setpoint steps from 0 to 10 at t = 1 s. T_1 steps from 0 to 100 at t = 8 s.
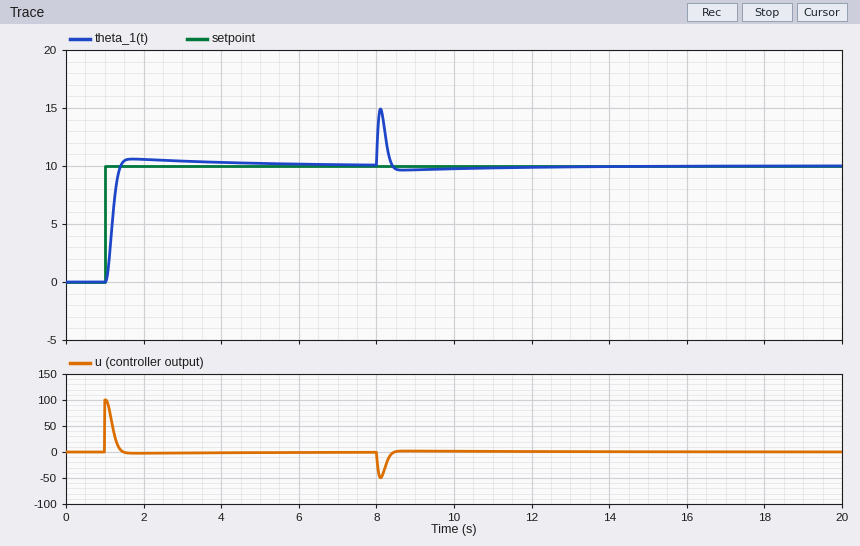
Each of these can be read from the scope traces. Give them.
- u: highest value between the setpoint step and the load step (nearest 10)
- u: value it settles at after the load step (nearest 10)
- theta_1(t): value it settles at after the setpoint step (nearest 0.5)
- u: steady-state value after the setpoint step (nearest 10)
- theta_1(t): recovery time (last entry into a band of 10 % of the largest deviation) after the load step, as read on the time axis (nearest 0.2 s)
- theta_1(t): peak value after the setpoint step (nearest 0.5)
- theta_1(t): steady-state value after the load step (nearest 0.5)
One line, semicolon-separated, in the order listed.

100; 0; 10.0; 0; 8.4 s; 10.5; 10.0
